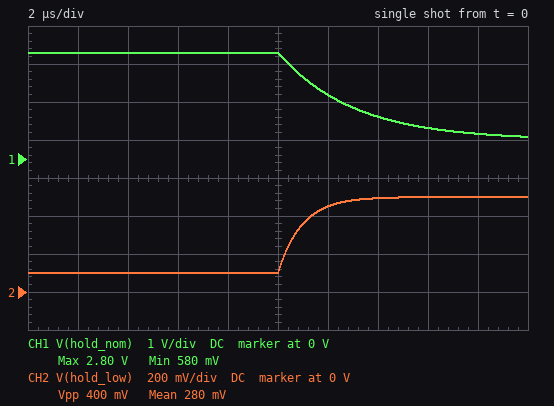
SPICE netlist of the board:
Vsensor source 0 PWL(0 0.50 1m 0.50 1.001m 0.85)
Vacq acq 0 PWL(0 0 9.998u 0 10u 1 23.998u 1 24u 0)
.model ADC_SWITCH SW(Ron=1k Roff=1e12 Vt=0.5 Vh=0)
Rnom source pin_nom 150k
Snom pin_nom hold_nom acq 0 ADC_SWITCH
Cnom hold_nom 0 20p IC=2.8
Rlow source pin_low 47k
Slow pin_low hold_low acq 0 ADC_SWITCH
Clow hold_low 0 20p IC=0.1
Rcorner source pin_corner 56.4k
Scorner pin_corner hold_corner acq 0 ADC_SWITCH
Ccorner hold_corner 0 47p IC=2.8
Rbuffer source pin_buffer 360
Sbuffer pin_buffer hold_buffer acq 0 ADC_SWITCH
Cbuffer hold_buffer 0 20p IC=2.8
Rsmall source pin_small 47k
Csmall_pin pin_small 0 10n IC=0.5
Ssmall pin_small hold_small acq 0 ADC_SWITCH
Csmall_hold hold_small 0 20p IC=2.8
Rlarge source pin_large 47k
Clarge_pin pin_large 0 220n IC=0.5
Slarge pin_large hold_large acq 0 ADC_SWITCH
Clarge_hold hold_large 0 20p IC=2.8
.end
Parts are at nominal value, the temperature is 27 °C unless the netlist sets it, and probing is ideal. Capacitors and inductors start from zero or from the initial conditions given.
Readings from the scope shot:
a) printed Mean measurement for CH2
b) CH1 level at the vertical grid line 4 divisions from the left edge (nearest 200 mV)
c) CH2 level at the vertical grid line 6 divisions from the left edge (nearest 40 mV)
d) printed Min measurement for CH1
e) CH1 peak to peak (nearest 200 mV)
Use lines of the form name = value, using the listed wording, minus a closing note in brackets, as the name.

printed Mean measurement for CH2 = 280 mV
CH1 level at the vertical grid line 4 divisions from the left edge = 2.8 V
CH2 level at the vertical grid line 6 divisions from the left edge = 440 mV
printed Min measurement for CH1 = 580 mV
CH1 peak to peak = 2.2 V
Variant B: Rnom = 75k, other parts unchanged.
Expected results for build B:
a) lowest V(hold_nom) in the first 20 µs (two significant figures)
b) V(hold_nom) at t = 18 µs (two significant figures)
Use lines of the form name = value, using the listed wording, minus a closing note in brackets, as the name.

lowest V(hold_nom) in the first 20 µs = 500 mV
V(hold_nom) at t = 18 µs = 510 mV
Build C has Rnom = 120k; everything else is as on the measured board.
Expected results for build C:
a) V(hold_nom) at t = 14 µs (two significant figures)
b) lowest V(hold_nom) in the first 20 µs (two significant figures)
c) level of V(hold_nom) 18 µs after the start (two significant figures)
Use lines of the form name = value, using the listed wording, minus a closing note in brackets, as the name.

V(hold_nom) at t = 14 µs = 940 mV
lowest V(hold_nom) in the first 20 µs = 540 mV
level of V(hold_nom) 18 µs after the start = 580 mV
